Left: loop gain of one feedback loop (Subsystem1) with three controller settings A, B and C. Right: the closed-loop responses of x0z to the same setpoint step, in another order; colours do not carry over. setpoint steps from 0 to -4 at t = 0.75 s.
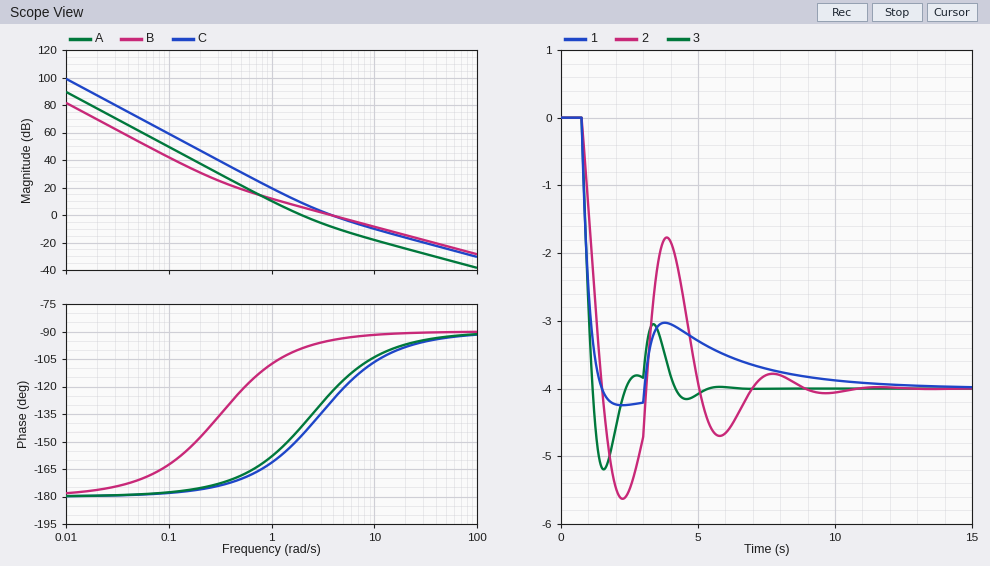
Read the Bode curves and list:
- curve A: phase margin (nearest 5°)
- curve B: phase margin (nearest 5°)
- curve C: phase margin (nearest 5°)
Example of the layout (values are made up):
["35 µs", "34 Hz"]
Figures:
["40°", "85°", "50°"]
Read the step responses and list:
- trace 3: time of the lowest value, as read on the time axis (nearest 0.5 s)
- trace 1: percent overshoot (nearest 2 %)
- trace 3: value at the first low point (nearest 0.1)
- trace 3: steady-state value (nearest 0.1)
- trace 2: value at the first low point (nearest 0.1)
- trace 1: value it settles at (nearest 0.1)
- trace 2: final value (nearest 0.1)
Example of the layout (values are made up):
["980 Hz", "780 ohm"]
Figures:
["1.5 s", "6 %", "-5.2", "-4.0", "-5.6", "-4.0", "-4.0"]
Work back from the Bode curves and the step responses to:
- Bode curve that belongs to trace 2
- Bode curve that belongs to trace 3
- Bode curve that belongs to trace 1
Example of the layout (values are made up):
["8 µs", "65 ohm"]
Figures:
["A", "C", "B"]
